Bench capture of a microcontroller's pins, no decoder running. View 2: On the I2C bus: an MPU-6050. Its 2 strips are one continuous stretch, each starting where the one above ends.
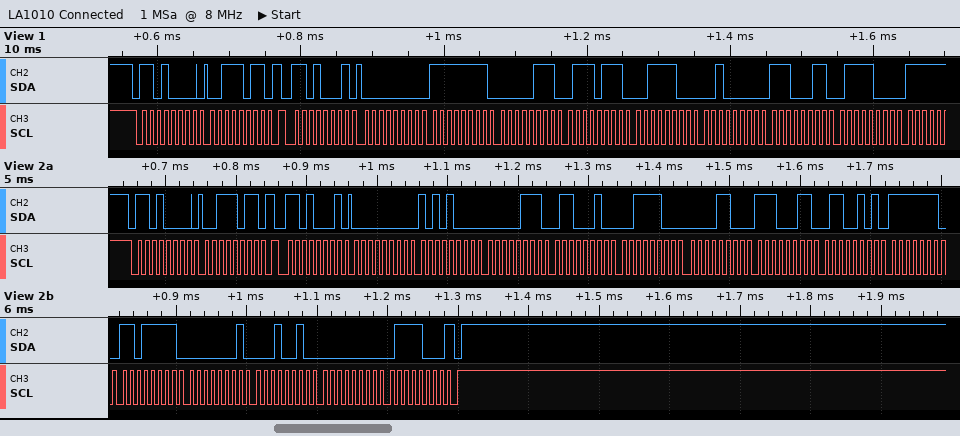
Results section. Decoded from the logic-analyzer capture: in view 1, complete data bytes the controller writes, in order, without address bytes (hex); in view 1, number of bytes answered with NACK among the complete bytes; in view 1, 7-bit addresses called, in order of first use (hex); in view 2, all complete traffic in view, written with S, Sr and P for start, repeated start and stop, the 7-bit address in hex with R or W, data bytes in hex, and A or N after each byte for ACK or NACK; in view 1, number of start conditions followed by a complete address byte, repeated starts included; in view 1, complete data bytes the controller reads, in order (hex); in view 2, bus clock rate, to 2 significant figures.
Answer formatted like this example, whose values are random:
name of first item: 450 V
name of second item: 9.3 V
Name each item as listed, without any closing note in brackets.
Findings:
in view 1, complete data bytes the controller writes, in order, without address bytes: 3B
in view 1, number of bytes answered with NACK among the complete bytes: 0
in view 1, 7-bit addresses called, in order of first use: 0x68
in view 2, all complete traffic in view, written with S, Sr and P for start, repeated start and stop, the 7-bit address in hex with R or W, data bytes in hex, and A or N after each byte for ACK or NACK: S 68W A 3B A Sr 68R A 00 A A8 A 07 A 62 A 3C A 0C A E3 A 65 A FE A DF A 01 A 12 A 00 A 78 N P
in view 1, number of start conditions followed by a complete address byte, repeated starts included: 2
in view 1, complete data bytes the controller reads, in order: 00 FF 07 77 3C 20 E3 78
in view 2, bus clock rate, to 2 significant figures: 100 kHz
